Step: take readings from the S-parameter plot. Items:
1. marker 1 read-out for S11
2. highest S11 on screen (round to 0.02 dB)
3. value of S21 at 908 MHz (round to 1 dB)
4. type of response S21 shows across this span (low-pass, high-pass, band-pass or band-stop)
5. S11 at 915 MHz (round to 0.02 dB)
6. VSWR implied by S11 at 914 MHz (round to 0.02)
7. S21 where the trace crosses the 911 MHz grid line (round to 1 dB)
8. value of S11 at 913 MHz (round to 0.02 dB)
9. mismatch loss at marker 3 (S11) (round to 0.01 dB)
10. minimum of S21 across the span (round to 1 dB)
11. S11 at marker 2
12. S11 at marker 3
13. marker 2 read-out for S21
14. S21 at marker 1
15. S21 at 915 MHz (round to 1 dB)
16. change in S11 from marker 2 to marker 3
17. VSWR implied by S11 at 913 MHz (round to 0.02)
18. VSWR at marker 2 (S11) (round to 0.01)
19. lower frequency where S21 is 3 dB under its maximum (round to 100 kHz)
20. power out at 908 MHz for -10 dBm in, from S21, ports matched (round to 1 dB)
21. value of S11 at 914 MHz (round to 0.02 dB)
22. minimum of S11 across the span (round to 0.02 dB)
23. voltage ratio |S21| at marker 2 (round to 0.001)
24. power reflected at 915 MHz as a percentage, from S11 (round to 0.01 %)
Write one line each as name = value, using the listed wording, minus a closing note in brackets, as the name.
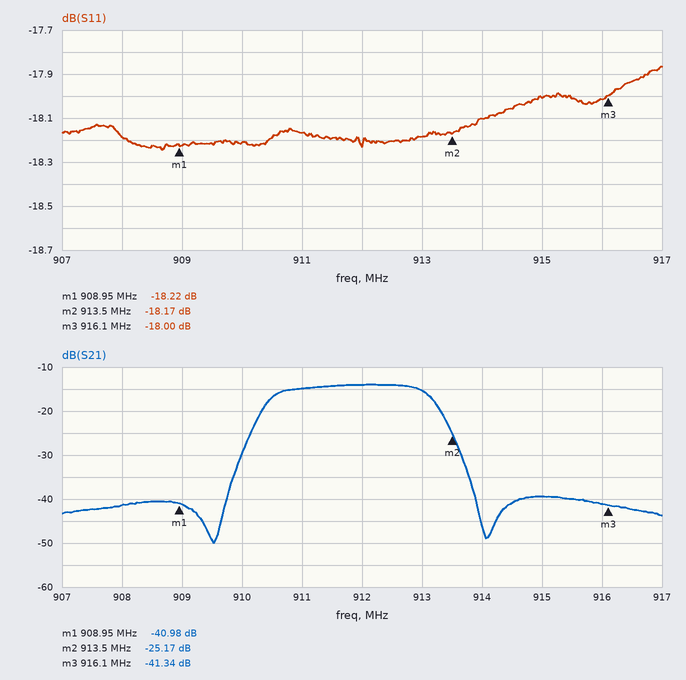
marker 1 read-out for S11 = -18.22 dB
highest S11 on screen = -17.86 dB
value of S21 at 908 MHz = -41 dB
type of response S21 shows across this span = band-pass
S11 at 915 MHz = -18.00 dB
VSWR implied by S11 at 914 MHz = 1.28
S21 where the trace crosses the 911 MHz grid line = -15 dB
value of S11 at 913 MHz = -18.18 dB
mismatch loss at marker 3 (S11) = 0.07 dB
minimum of S21 across the span = -50 dB
S11 at marker 2 = -18.17 dB
S11 at marker 3 = -18.00 dB
marker 2 read-out for S21 = -25.17 dB
S21 at marker 1 = -40.98 dB
S21 at 915 MHz = -39 dB
change in S11 from marker 2 to marker 3 = 0.17 dB
VSWR implied by S11 at 913 MHz = 1.28
VSWR at marker 2 (S11) = 1.28
lower frequency where S21 is 3 dB under its maximum = 910.5 MHz
power out at 908 MHz for -10 dBm in, from S21, ports matched = -51 dBm
value of S11 at 914 MHz = -18.10 dB
minimum of S11 across the span = -18.24 dB
voltage ratio |S21| at marker 2 = 0.055
power reflected at 915 MHz as a percentage, from S11 = 1.58 %
